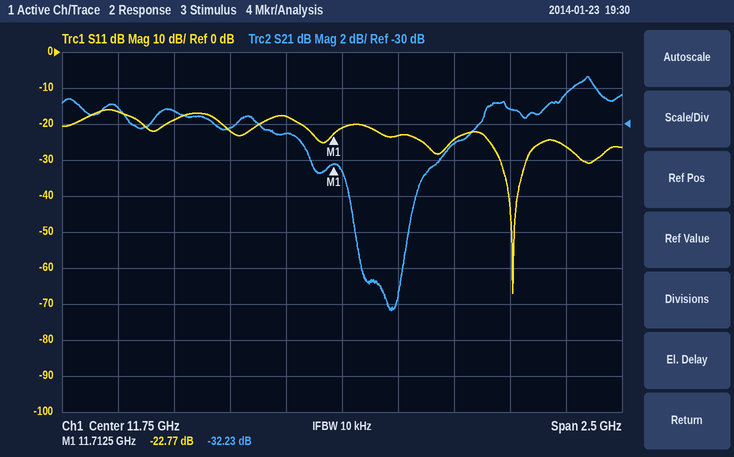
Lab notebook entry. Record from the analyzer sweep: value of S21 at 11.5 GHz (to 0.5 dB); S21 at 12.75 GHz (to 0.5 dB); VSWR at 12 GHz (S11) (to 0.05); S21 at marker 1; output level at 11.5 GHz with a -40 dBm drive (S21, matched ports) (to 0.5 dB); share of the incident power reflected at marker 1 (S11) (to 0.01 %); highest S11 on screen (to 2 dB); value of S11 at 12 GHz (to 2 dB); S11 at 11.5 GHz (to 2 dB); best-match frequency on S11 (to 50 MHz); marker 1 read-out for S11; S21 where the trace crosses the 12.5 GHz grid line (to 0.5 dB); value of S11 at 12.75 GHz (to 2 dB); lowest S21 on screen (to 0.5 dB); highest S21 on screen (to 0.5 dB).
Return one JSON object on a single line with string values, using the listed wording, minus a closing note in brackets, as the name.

{"value of S21 at 11.5 GHz": "-30.5 dB", "S21 at 12.75 GHz": "-28.5 dB", "VSWR at 12 GHz (S11)": "1.15", "S21 at marker 1": "-32.23 dB", "output level at 11.5 GHz with a -40 dBm drive (S21, matched ports)": "-70.5 dBm", "share of the incident power reflected at marker 1 (S11)": "0.53 %", "highest S11 on screen": "-16 dB", "value of S11 at 12 GHz": "-24 dB", "S11 at 11.5 GHz": "-18 dB", "best-match frequency on S11": "12.50 GHz", "marker 1 read-out for S11": "-22.77 dB", "S21 where the trace crosses the 12.5 GHz grid line": "-29.0 dB", "value of S11 at 12.75 GHz": "-26 dB", "lowest S21 on screen": "-40.5 dB", "highest S21 on screen": "-27.5 dB"}
